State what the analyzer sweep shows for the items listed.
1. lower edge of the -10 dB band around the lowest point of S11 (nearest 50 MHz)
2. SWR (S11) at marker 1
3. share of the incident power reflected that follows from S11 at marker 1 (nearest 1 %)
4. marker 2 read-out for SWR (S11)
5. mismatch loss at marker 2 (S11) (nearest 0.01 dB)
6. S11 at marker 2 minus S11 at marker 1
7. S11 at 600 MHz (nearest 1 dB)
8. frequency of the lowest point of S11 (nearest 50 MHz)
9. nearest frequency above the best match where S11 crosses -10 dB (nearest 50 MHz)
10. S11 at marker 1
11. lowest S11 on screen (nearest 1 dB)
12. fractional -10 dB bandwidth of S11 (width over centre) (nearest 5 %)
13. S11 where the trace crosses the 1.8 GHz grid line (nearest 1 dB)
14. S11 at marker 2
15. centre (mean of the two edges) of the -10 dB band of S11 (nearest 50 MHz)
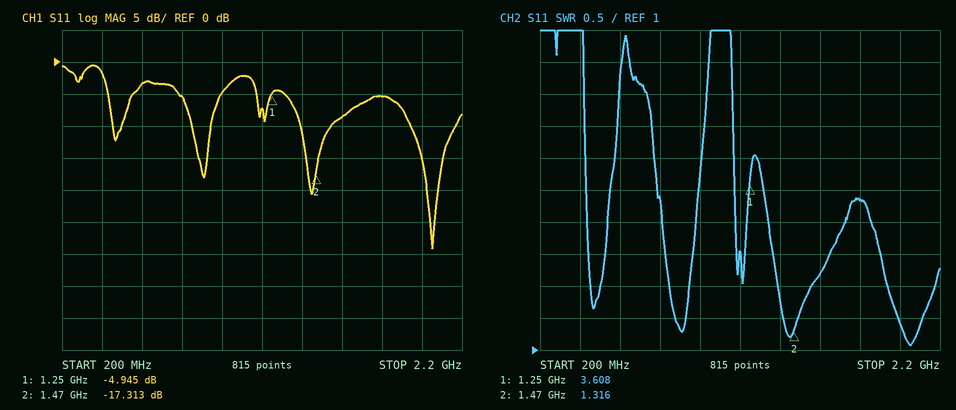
1.95 GHz
3.608
32 %
1.316
0.08 dB
-12.368 dB
-3 dB
2.05 GHz
2.15 GHz
-4.945 dB
-29 dB
10 %
-5 dB
-17.313 dB
2.05 GHz
